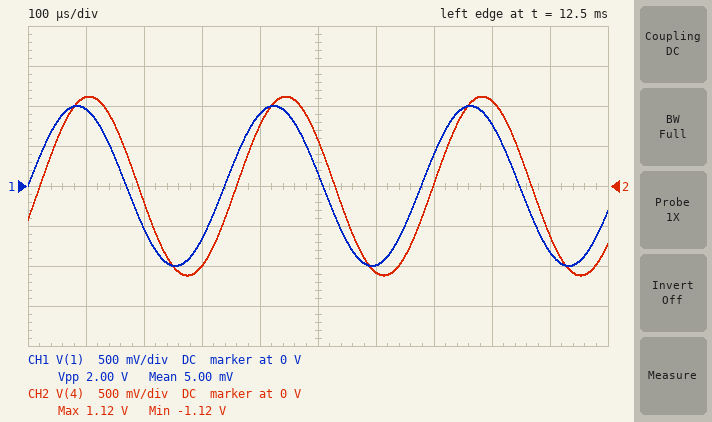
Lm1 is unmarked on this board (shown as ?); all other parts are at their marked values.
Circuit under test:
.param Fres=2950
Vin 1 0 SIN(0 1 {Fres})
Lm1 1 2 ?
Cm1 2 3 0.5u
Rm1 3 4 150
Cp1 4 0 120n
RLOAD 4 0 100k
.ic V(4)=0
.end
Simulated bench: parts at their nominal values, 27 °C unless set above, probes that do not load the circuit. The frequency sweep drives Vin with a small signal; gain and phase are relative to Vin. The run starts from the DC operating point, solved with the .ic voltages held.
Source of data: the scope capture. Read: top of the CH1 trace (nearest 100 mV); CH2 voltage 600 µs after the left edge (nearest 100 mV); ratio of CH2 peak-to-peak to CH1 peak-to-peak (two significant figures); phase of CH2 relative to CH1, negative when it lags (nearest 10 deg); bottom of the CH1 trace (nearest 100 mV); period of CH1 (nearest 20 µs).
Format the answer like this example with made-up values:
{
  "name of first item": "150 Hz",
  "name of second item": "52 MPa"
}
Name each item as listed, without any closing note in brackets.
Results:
{
  "top of the CH1 trace": "1.0 V",
  "CH2 voltage 600 µs after the left edge": "-1.1 V",
  "ratio of CH2 peak-to-peak to CH1 peak-to-peak": "1.1",
  "phase of CH2 relative to CH1, negative when it lags": "-20 deg",
  "bottom of the CH1 trace": "-1.0 V",
  "period of CH1": "340 µs"
}
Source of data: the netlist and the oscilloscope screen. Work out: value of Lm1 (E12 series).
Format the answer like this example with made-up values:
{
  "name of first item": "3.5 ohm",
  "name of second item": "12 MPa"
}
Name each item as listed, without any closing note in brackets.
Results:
{
  "value of Lm1": "10 mH"
}
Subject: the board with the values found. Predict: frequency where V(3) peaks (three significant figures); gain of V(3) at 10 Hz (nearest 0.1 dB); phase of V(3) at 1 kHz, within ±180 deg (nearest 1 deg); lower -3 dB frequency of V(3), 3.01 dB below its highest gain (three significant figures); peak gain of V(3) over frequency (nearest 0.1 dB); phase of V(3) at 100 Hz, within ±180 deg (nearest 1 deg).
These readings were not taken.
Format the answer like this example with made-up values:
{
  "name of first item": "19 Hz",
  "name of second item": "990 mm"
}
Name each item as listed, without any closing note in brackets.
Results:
{
  "frequency where V(3) peaks": "4.90 kHz",
  "gain of V(3) at 10 Hz": "-2.1 dB",
  "phase of V(3) at 1 kHz, within ±180 deg": "1 deg",
  "lower -3 dB frequency of V(3), 3.01 dB below its highest gain": "3.57 kHz",
  "peak gain of V(3) over frequency": "6.1 dB",
  "phase of V(3) at 100 Hz, within ±180 deg": "2 deg"
}
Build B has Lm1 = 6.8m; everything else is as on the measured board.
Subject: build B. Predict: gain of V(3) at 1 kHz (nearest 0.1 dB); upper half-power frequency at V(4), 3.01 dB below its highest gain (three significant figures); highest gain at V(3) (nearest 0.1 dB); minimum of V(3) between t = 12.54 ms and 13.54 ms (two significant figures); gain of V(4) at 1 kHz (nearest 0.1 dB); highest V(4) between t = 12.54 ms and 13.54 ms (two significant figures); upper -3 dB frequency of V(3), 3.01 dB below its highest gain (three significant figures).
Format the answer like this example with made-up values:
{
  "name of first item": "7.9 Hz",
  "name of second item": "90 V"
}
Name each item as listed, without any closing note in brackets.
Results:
{
  "gain of V(3) at 1 kHz": "-1.6 dB",
  "upper half-power frequency at V(4), 3.01 dB below its highest gain": "7.30 kHz",
  "highest gain at V(3)": "5.0 dB",
  "minimum of V(3) between t = 12.54 ms and 13.54 ms": "-1.0 V",
  "gain of V(4) at 1 kHz": "-1.7 dB",
  "highest V(4) between t = 12.54 ms and 13.54 ms": "980 mV",
  "upper -3 dB frequency of V(3), 3.01 dB below its highest gain": "7.58 kHz"
}
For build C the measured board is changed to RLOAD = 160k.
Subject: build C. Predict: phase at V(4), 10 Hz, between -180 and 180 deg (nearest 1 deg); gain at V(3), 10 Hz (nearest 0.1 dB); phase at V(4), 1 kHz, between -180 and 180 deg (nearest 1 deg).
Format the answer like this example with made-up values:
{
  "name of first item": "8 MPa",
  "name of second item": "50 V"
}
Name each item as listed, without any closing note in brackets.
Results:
{
  "phase at V(4), 10 Hz, between -180 and 180 deg": "9 deg",
  "gain at V(3), 10 Hz": "-2.0 dB",
  "phase at V(4), 1 kHz, between -180 and 180 deg": "-5 deg"
}
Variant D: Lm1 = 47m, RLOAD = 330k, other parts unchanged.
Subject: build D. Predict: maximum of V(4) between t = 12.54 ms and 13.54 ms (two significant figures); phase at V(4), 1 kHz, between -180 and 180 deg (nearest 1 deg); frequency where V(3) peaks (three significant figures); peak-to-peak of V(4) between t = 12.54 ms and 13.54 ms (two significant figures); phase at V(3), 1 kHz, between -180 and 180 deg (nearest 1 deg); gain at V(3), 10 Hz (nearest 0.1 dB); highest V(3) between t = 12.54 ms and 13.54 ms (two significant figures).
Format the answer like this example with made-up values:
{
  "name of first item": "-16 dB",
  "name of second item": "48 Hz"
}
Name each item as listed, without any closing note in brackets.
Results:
{
  "maximum of V(4) between t = 12.54 ms and 13.54 ms": "1.3 V",
  "phase at V(4), 1 kHz, between -180 and 180 deg": "-6 deg",
  "frequency where V(3) peaks": "2.33 kHz",
  "peak-to-peak of V(4) between t = 12.54 ms and 13.54 ms": "2.6 V",
  "phase at V(3), 1 kHz, between -180 and 180 deg": "0 deg",
  "gain at V(3), 10 Hz": "-1.9 dB",
  "highest V(3) between t = 12.54 ms and 13.54 ms": "1.4 V"
}
